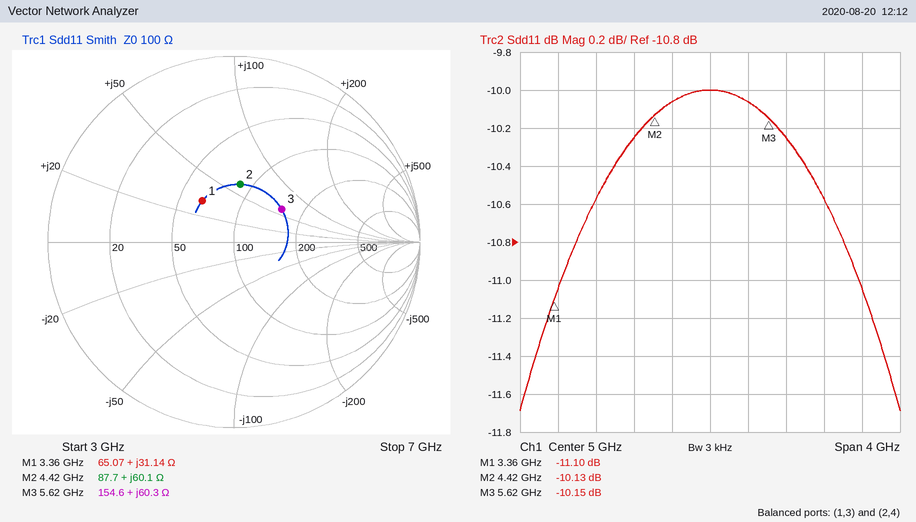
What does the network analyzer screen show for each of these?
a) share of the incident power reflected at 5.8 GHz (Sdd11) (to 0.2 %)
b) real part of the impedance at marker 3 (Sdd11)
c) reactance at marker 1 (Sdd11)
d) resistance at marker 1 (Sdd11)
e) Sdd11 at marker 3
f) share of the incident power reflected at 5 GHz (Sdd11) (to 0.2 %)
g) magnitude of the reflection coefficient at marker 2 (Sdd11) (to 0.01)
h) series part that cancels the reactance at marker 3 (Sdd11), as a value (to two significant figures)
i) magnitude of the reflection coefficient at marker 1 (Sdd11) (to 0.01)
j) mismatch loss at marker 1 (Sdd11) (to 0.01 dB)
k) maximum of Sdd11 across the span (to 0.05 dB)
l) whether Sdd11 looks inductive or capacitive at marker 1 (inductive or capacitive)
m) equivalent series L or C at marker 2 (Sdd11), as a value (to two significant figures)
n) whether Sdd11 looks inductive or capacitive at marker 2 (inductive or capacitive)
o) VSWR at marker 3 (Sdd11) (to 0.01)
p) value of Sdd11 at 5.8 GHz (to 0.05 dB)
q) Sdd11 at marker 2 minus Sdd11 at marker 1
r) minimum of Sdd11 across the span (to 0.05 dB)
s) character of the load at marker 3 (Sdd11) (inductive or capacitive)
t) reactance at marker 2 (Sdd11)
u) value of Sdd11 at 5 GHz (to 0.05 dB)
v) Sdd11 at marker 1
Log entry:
9.4 %
154.6 Ω
+31.14 Ω
65.07 Ω
-10.15 dB
10.0 %
0.31
470 fF
0.28
0.35 dB
-10.00 dB
inductive
2.2 nH
inductive
1.90
-10.25 dB
0.97 dB
-11.70 dB
inductive
+60.1 Ω
-10.00 dB
-11.10 dB
